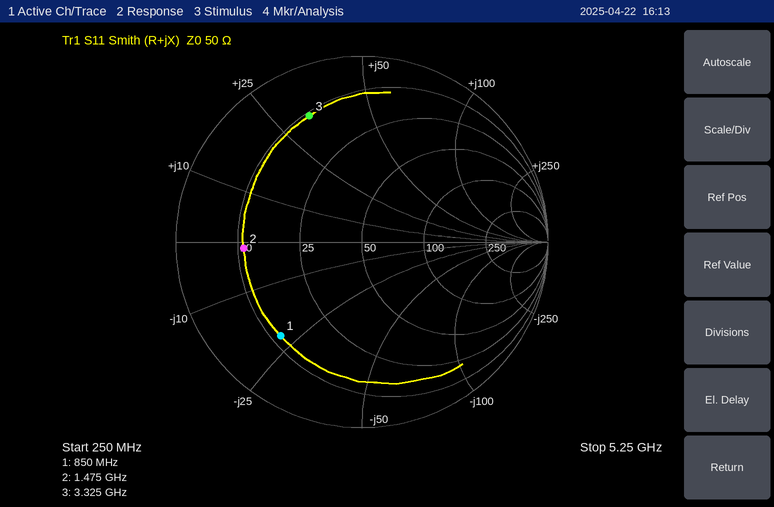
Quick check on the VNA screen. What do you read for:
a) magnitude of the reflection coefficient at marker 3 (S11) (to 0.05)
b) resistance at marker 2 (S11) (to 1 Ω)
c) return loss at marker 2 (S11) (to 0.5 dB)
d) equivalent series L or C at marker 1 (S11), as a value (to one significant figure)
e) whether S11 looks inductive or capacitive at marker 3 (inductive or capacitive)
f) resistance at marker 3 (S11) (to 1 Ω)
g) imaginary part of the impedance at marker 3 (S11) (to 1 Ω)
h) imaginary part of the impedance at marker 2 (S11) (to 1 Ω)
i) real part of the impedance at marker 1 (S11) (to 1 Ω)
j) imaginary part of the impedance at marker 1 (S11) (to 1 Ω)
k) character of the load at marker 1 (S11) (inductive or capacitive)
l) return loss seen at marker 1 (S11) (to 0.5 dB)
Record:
0.75
11 Ω
4.0 dB
9 pF
inductive
11 Ω
+32 Ω
-1 Ω
12 Ω
-22 Ω
capacitive
3.5 dB
